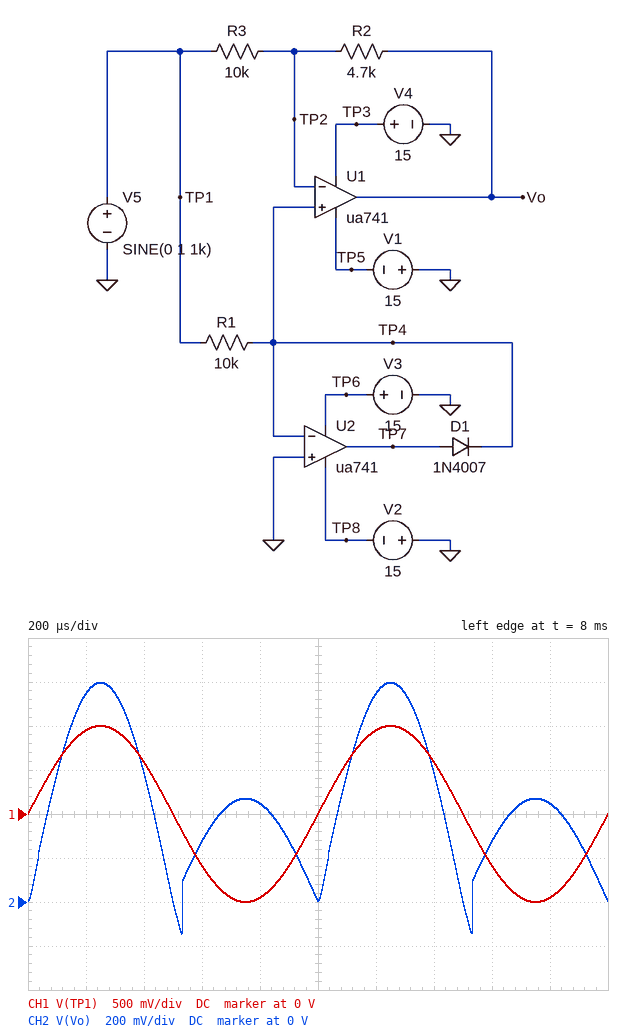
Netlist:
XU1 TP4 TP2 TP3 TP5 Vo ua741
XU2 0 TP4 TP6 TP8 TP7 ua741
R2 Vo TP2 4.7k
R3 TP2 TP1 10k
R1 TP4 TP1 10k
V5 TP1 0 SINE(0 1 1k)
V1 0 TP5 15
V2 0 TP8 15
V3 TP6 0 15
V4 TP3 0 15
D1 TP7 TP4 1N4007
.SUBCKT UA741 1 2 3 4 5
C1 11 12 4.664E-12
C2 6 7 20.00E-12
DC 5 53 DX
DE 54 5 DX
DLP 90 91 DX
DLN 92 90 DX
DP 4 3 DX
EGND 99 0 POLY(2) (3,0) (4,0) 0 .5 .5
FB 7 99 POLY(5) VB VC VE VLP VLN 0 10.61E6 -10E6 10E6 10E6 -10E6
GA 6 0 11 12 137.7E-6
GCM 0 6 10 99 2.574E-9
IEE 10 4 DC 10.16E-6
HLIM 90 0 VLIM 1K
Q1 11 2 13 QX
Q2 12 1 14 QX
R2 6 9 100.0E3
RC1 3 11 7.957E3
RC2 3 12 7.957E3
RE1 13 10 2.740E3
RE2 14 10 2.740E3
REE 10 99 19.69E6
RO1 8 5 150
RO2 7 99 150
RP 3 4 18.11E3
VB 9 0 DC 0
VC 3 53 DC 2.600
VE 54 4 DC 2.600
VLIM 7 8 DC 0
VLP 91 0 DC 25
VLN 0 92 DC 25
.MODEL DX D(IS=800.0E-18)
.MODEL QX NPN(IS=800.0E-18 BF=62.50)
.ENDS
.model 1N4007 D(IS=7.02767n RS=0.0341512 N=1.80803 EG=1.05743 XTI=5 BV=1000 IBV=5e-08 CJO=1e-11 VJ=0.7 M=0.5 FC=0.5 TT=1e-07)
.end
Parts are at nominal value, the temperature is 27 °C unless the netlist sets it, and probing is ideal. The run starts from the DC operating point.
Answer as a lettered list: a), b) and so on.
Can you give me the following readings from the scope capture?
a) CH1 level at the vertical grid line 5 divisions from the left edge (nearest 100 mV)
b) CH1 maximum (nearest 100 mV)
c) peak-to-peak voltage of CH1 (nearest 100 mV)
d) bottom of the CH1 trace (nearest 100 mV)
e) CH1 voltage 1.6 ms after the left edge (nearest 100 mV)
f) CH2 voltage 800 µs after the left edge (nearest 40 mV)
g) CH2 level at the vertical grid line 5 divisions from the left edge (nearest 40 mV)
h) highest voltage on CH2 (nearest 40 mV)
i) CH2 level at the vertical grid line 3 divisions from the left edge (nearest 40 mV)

a) 0 V
b) 1.0 V
c) 2.0 V
d) -1.0 V
e) -600 mV
f) 440 mV
g) 0 V
h) 1.00 V
i) 280 mV
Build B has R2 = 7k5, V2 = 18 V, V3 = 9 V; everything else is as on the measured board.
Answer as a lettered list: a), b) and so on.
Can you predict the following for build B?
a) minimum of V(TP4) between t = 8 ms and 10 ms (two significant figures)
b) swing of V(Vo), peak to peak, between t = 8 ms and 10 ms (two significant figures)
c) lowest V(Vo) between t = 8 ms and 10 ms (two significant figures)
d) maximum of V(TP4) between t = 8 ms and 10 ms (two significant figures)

a) -190 mV
b) 1.2 V
c) -160 mV
d) 1.0 V
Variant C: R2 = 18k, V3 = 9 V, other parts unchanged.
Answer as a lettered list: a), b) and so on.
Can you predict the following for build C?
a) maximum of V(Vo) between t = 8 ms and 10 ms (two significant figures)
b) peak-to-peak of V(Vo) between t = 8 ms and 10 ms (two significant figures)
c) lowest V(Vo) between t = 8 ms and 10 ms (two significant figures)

a) 1.8 V
b) 1.9 V
c) -100 mV
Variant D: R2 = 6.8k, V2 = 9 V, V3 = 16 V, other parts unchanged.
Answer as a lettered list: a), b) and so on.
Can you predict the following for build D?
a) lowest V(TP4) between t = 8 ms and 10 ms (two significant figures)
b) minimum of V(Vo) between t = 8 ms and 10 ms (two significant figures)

a) -97 mV
b) -76 mV
